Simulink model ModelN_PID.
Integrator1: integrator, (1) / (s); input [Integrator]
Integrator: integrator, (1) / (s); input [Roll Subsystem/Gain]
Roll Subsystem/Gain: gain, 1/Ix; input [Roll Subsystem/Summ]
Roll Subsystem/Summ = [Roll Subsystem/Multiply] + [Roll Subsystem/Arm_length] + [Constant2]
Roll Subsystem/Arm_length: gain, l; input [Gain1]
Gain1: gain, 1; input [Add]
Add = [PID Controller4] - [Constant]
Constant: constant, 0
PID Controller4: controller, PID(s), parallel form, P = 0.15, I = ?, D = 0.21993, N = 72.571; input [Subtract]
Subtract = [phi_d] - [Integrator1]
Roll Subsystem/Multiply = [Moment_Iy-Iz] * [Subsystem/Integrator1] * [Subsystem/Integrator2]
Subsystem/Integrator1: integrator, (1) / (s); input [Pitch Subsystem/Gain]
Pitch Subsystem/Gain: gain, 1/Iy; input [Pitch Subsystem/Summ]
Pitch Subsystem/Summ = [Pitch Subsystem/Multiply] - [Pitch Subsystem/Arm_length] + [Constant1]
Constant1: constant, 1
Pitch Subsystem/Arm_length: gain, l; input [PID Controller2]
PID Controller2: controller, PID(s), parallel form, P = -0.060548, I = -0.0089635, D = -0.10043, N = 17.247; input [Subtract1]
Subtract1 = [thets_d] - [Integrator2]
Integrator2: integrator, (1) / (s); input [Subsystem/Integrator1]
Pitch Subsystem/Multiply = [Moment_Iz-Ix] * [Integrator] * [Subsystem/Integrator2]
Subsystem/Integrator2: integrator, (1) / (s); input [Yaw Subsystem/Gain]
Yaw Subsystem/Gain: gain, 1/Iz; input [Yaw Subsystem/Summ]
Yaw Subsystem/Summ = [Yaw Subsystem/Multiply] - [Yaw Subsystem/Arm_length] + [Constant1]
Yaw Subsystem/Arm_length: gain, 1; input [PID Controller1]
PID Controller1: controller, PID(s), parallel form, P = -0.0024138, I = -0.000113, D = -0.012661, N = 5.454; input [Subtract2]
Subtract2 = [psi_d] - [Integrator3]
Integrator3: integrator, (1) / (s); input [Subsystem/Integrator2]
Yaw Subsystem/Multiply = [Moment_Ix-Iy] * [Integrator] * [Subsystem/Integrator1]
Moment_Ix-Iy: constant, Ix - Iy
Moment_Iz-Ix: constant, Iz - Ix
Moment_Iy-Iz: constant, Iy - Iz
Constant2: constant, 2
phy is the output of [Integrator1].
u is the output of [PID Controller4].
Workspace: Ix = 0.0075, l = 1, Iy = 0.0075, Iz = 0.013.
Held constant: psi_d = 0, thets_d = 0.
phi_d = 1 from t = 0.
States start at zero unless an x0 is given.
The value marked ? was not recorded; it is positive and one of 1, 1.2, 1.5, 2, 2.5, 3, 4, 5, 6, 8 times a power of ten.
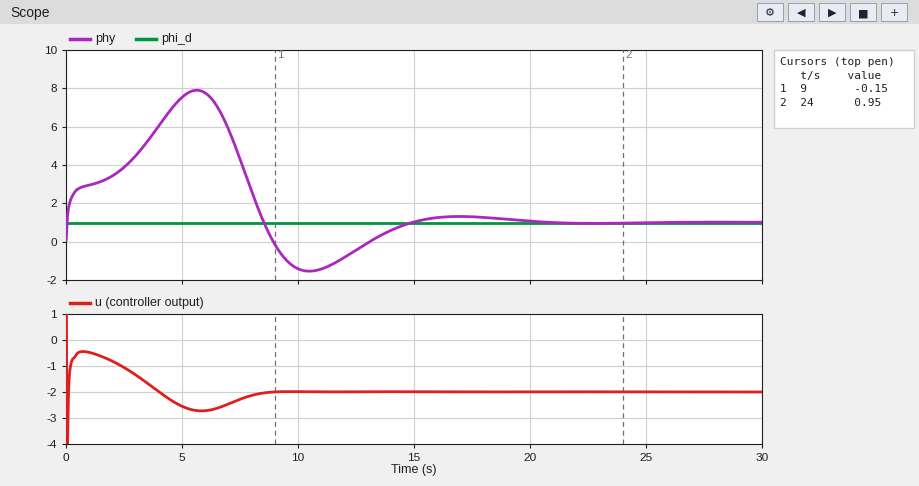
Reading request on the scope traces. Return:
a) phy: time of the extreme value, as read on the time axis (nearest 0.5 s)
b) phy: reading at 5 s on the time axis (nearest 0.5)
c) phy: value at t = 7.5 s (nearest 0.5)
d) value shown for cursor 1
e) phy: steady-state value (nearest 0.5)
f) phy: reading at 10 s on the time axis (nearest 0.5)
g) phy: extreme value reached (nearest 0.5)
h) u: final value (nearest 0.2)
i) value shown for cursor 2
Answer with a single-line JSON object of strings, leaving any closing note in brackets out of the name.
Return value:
{"phy: time of the extreme value, as read on the time axis": "5.5 s", "phy: reading at 5 s on the time axis": "7.5", "phy: value at t = 7.5 s": "4.5", "value shown for cursor 1": "-0.15", "phy: steady-state value": "1.0", "phy: reading at 10 s on the time axis": "-1.5", "phy: extreme value reached": "8.0", "u: final value": "-2.0", "value shown for cursor 2": "0.95"}
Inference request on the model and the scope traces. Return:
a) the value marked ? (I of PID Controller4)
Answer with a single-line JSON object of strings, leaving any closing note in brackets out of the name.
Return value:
{"the value marked ?": "0.08"}
